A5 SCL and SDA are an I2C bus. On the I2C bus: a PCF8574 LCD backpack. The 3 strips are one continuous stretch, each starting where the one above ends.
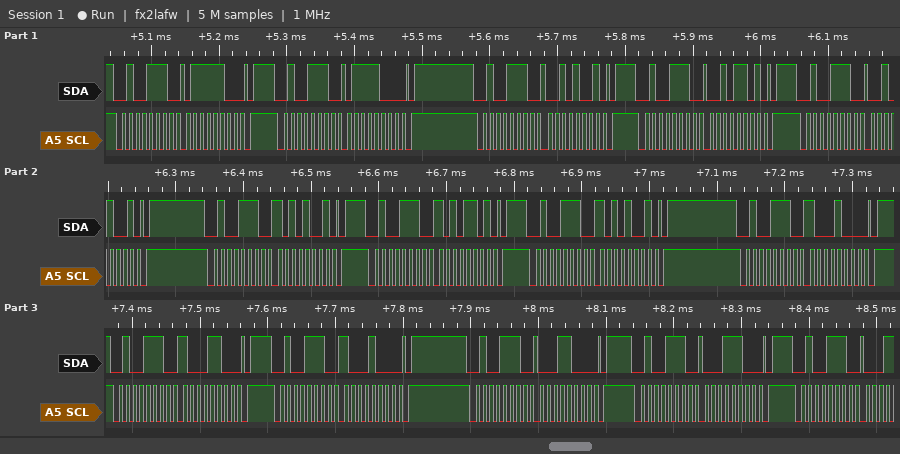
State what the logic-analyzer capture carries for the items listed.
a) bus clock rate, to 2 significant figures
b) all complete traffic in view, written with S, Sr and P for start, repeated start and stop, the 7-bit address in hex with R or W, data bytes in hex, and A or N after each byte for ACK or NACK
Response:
100 kHz
S 27W A 7C A P S 27W A 78 A P S 27W A 29 A P S 27W A 2D A P S 27W A 29 A P S 27W A A9 A P S 27W A AD A P S 27W A A9 A P S 27W A 88 A P S 27W A 8C A P S 27W A 88 A P S 27W A 18 A P S 27W A 1C A P S 27W A
